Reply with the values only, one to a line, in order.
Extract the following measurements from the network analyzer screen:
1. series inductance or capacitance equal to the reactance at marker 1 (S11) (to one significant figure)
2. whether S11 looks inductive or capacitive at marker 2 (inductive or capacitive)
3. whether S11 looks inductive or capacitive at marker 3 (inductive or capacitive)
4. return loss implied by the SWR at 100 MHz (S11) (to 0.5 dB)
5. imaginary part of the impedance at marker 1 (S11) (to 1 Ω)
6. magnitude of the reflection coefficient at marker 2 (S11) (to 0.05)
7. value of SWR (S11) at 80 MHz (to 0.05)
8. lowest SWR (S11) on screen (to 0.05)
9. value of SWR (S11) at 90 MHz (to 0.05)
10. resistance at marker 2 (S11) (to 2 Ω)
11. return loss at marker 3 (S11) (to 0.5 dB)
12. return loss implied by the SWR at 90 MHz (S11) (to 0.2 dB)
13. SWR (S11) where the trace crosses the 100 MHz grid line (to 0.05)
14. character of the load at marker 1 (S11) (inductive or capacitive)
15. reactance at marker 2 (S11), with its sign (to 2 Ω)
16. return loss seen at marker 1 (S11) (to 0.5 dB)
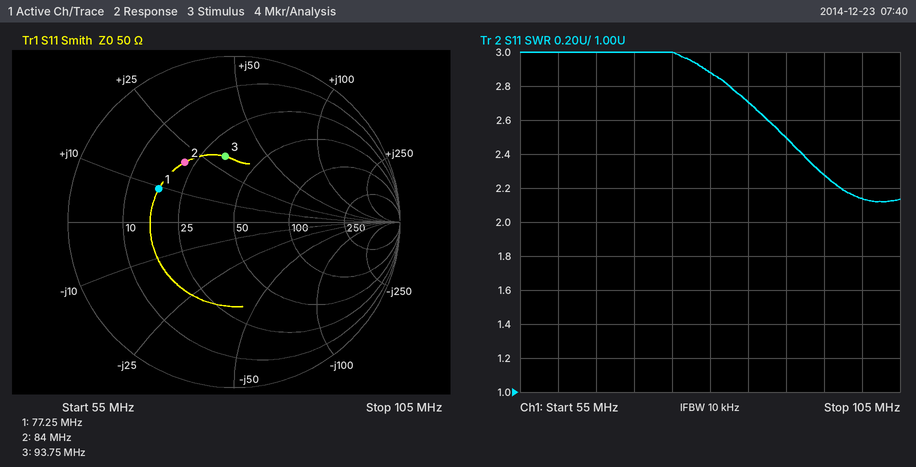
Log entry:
20 nH
inductive
inductive
9.0 dB
+9 Ω
0.45
2.90
2.10
2.50
22 Ω
8.0 dB
7.4 dB
2.15
inductive
+20 Ω
6.0 dB
